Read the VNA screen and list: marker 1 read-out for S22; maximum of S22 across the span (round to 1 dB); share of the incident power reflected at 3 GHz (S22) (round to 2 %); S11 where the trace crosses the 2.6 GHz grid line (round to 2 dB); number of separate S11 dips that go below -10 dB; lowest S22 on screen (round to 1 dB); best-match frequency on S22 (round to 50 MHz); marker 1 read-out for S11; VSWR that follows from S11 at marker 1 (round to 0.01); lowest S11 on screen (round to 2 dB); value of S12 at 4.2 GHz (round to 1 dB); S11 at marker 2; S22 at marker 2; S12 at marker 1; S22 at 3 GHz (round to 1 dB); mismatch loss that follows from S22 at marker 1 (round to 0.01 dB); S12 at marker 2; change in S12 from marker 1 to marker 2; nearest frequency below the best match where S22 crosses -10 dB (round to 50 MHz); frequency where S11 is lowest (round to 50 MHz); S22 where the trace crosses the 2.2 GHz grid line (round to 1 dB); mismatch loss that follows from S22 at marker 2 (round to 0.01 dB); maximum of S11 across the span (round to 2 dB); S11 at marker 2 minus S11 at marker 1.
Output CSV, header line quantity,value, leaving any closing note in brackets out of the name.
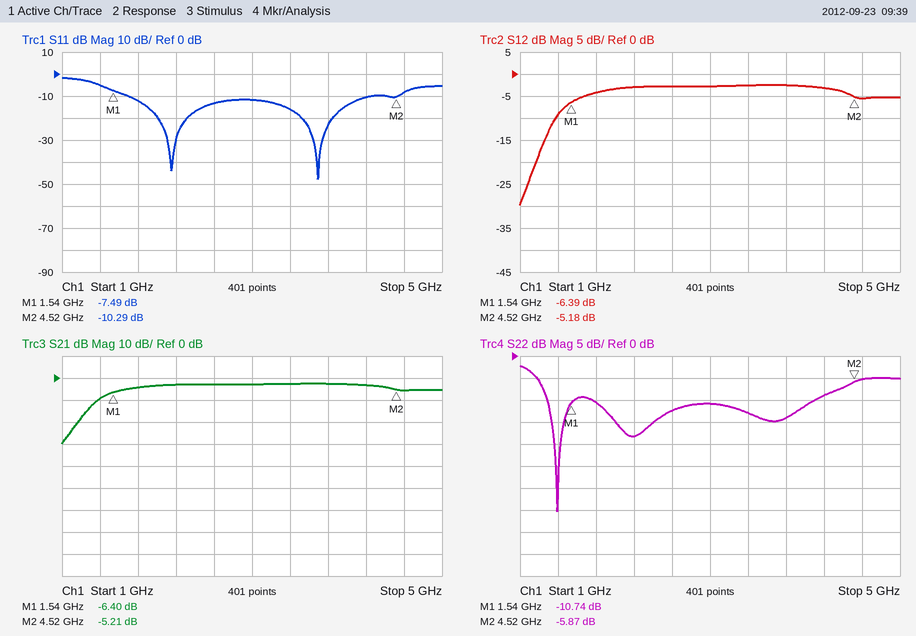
quantity,value
marker 1 read-out for S22,-10.74 dB
maximum of S22 across the span,-2 dB
share of the incident power reflected at 3 GHz (S22),8 %
S11 where the trace crosses the 2.6 GHz grid line,-14 dB
number of separate S11 dips that go below -10 dB,2
lowest S22 on screen,-35 dB
best-match frequency on S22,1.40 GHz
marker 1 read-out for S11,-7.49 dB
VSWR that follows from S11 at marker 1,2.46
lowest S11 on screen,-48 dB
value of S12 at 4.2 GHz,-3 dB
S11 at marker 2,-10.29 dB
S22 at marker 2,-5.87 dB
S12 at marker 1,-6.39 dB
S22 at 3 GHz,-11 dB
mismatch loss that follows from S22 at marker 1,0.38 dB
S12 at marker 2,-5.18 dB
change in S12 from marker 1 to marker 2,1.21 dB
nearest frequency below the best match where S22 crosses -10 dB,1.30 GHz
frequency where S11 is lowest,3.70 GHz
S22 where the trace crosses the 2.2 GHz grid line,-18 dB
mismatch loss that follows from S22 at marker 2,1.30 dB
maximum of S11 across the span,-2 dB
S11 at marker 2 minus S11 at marker 1,-2.80 dB
